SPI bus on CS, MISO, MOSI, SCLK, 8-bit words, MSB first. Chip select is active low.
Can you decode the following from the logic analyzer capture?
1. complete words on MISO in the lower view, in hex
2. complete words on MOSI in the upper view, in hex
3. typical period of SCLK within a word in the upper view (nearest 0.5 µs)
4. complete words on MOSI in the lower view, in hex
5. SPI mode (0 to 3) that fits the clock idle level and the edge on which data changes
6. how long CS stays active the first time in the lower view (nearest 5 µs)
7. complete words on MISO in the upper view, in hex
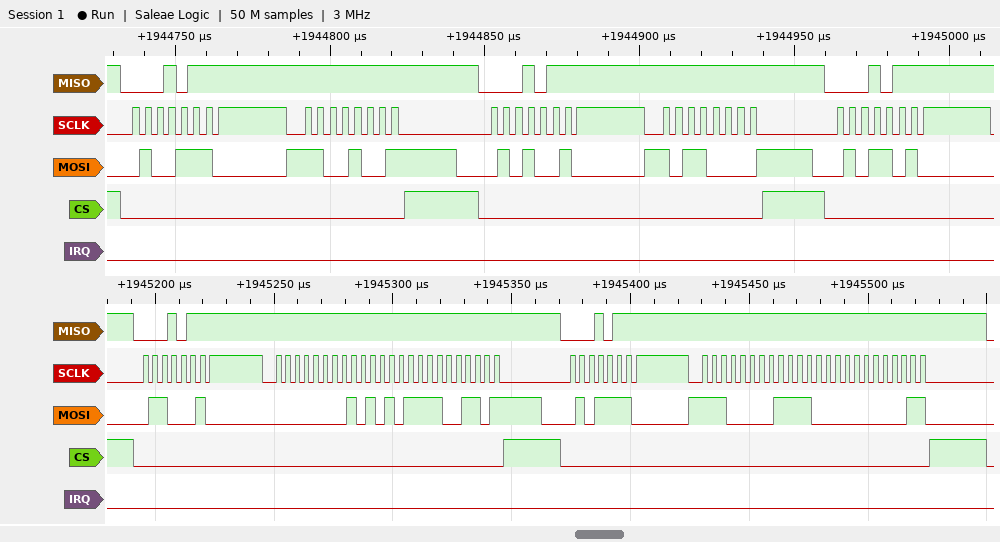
17, FF, FF, FF, 17, FF, FF, FF
4E, C9, 52, B0, 5A
4 µs
62, 00, AB, CD, 5E, E0, F0, 03
0
155 µs
17, FF, 17, FF, 17
